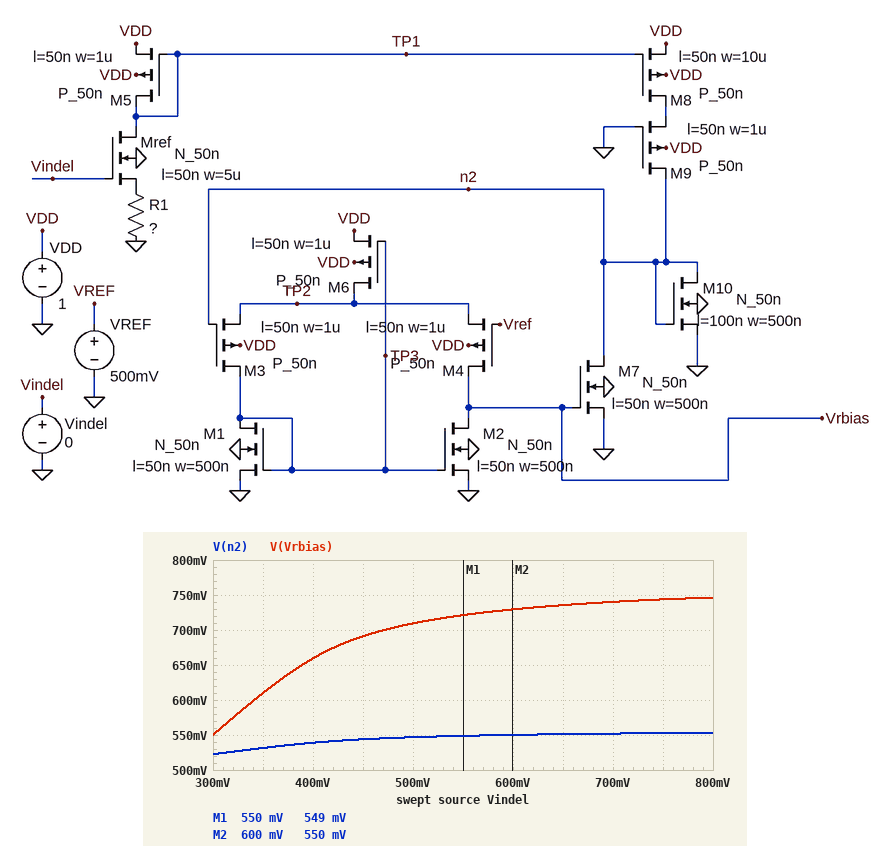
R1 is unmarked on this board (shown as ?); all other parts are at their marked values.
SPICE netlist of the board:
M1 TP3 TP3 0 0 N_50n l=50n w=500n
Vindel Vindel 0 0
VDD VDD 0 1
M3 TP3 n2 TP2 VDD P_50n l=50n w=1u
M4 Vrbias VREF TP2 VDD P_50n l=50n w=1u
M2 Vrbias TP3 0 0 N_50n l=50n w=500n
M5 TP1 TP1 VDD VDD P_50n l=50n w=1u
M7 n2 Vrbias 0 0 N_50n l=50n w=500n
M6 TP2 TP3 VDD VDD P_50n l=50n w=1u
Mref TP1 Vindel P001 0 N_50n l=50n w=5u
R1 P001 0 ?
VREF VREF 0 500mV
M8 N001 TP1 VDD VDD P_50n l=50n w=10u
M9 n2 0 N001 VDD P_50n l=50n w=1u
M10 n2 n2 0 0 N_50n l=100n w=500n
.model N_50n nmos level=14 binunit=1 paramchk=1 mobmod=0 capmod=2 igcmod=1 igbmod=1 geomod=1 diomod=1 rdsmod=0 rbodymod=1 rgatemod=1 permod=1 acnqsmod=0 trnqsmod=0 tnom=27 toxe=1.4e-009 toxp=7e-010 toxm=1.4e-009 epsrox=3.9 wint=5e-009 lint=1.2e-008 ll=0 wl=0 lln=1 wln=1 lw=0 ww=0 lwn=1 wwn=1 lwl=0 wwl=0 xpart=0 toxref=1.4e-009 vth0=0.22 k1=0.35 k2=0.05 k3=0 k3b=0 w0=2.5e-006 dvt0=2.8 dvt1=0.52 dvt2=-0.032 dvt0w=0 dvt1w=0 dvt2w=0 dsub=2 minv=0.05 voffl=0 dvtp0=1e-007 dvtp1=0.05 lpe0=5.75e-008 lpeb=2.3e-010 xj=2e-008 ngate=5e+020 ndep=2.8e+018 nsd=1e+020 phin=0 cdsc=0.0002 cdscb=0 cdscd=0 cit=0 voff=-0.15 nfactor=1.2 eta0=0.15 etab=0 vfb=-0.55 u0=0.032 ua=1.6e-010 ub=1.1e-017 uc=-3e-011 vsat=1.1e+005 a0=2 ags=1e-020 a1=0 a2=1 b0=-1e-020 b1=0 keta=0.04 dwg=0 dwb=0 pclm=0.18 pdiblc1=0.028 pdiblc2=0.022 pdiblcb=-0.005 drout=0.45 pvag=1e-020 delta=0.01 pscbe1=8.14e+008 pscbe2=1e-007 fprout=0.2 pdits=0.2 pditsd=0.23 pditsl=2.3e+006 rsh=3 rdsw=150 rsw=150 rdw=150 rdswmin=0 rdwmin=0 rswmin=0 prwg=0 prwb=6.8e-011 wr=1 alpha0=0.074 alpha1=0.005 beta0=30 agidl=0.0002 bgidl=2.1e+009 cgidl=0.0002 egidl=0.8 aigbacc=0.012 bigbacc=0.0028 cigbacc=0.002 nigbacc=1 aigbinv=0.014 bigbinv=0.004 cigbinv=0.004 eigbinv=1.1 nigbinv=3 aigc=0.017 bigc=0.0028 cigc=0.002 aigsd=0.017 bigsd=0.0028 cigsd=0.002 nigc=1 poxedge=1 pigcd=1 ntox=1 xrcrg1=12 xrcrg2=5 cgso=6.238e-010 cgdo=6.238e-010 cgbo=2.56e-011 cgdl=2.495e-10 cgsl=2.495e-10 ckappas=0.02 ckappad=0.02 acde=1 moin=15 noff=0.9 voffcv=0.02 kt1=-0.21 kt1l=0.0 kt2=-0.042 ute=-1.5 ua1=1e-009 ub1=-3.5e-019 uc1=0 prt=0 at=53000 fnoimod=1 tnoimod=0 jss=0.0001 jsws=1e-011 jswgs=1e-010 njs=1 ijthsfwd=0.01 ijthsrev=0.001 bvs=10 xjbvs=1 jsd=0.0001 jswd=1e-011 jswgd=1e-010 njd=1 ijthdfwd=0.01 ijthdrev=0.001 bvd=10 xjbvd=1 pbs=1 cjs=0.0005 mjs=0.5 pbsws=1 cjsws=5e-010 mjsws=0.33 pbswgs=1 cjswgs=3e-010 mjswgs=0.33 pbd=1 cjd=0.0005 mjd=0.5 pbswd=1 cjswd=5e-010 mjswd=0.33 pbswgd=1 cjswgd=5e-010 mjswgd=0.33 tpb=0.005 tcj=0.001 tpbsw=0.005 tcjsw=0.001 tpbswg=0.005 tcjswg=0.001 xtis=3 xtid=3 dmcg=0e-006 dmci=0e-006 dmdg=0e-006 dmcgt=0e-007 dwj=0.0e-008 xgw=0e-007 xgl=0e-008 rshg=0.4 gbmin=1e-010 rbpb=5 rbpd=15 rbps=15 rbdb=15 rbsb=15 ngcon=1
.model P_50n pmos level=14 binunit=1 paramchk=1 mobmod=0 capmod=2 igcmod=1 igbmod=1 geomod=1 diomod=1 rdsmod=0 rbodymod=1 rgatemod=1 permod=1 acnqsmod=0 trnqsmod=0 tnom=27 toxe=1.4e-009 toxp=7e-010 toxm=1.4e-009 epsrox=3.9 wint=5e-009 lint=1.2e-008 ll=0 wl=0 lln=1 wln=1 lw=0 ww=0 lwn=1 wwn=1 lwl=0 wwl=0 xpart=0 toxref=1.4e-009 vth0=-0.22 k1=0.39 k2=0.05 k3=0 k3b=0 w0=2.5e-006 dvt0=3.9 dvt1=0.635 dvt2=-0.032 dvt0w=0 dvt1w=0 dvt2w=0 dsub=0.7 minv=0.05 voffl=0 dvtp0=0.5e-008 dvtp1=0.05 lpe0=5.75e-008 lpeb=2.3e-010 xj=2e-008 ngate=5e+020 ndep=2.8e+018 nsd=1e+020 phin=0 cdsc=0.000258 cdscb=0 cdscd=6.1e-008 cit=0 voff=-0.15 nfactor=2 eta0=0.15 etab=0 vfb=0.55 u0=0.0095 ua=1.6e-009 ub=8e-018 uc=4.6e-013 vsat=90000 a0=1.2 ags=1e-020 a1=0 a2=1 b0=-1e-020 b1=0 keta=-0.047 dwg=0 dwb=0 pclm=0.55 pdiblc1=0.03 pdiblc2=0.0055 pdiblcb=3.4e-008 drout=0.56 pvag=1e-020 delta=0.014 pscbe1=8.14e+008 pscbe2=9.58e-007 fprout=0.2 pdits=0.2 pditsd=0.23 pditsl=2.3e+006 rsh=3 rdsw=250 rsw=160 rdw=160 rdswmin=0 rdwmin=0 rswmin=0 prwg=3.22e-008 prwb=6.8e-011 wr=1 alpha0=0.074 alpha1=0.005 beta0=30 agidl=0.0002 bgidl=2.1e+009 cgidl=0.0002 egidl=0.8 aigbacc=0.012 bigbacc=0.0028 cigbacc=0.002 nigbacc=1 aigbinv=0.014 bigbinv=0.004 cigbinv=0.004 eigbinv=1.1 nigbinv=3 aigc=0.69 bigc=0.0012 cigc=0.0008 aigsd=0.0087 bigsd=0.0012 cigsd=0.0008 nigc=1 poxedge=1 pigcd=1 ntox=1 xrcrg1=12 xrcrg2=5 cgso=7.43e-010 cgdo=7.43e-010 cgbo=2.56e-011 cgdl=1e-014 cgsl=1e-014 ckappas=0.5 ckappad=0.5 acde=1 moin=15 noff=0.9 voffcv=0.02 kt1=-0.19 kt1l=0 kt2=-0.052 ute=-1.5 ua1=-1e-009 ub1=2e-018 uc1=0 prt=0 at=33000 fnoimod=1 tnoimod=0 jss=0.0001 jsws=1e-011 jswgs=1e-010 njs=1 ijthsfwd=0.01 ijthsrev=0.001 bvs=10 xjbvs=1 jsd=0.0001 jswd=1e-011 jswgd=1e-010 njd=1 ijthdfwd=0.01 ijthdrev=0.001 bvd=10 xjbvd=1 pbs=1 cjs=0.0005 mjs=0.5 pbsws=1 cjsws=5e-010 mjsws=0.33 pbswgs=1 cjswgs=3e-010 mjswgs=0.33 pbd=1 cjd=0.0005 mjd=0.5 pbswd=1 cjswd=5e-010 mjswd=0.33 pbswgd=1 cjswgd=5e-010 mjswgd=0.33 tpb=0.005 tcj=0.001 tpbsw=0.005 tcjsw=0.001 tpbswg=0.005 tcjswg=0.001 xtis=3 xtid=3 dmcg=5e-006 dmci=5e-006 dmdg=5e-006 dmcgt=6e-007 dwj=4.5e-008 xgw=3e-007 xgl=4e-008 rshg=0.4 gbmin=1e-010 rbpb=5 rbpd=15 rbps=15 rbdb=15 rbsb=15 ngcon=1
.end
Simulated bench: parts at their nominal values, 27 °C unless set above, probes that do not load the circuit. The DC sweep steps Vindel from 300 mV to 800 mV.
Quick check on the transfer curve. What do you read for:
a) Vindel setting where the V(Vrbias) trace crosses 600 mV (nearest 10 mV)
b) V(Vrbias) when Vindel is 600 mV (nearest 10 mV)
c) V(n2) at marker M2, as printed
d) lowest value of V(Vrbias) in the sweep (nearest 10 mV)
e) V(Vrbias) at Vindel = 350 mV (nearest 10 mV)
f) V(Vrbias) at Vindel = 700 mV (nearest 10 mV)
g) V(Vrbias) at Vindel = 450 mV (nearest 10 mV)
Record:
340 mV
730 mV
550 mV
550 mV
610 mV
740 mV
690 mV
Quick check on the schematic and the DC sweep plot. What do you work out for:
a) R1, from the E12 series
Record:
5.6 kΩ
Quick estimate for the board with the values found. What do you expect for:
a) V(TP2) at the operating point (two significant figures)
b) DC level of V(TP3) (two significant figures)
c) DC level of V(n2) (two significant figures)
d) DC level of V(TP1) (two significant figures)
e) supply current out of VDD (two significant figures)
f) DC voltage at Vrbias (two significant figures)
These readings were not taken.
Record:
830 mV
460 mV
320 mV
870 mV
43 µA
16 mV
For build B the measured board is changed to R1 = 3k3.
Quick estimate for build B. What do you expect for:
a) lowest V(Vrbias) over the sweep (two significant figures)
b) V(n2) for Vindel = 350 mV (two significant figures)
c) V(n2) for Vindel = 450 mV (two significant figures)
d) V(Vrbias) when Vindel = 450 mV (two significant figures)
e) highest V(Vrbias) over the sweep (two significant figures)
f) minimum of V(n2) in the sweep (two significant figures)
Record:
600 mV
540 mV
550 mV
720 mV
760 mV
530 mV
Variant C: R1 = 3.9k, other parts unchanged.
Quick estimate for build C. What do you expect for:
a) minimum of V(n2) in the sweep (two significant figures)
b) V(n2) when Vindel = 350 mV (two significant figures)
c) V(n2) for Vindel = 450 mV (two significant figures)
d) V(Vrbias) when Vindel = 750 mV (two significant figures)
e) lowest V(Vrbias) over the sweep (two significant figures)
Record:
530 mV
540 mV
550 mV
750 mV
580 mV
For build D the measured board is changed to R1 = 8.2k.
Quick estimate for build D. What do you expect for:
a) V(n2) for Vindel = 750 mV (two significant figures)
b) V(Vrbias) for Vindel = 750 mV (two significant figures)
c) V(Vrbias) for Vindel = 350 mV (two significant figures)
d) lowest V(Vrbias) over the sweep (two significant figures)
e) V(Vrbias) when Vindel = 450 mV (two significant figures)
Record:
550 mV
730 mV
570 mV
520 mV
650 mV
